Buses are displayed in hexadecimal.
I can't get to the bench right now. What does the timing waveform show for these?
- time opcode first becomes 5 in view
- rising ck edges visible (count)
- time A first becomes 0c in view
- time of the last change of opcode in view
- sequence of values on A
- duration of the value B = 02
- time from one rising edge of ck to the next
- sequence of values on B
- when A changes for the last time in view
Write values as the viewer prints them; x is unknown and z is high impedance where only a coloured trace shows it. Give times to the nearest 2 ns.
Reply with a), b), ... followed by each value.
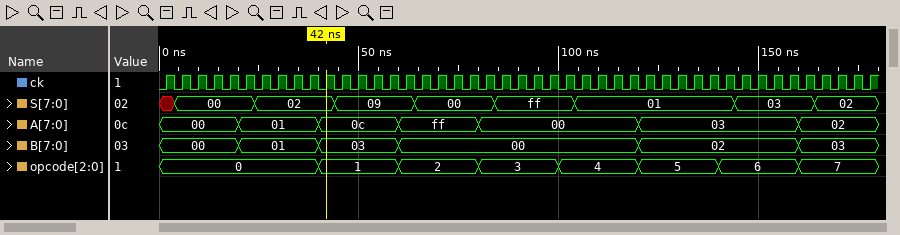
a) 120 ns
b) 45
c) 40 ns
d) 160 ns
e) 00, 01, 0c, ff, 00, 03, 02
f) 40 ns
g) 4 ns
h) 00, 01, 03, 00, 02, 03
i) 160 ns
